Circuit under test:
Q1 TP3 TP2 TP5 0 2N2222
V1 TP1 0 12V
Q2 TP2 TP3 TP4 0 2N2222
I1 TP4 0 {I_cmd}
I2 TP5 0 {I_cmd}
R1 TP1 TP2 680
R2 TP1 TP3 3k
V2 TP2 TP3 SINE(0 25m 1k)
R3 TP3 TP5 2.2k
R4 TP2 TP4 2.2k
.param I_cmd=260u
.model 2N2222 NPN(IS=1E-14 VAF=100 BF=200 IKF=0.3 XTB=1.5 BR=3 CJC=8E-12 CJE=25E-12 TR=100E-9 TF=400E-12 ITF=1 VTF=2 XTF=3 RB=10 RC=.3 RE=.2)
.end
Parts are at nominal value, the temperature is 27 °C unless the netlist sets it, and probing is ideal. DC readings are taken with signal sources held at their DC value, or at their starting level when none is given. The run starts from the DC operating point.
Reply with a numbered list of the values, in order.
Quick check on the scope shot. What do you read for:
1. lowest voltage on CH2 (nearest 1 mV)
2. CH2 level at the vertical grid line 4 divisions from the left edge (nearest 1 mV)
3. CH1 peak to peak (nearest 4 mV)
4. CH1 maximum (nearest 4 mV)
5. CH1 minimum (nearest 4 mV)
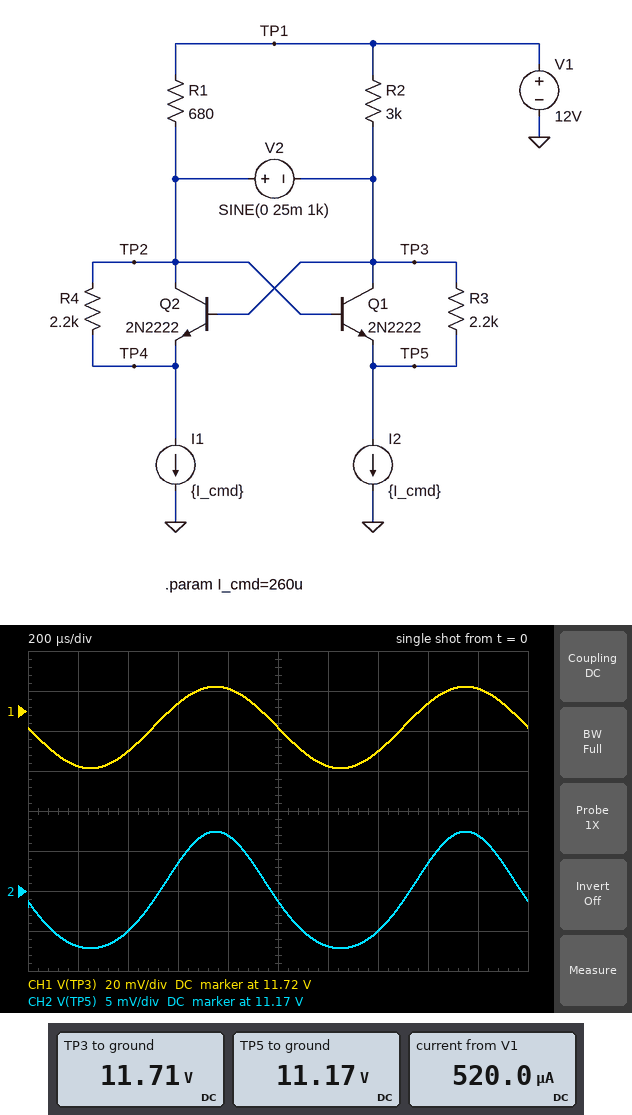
1. 11.163 V
2. 11.177 V
3. 40 mV
4. 11.732 V
5. 11.692 V
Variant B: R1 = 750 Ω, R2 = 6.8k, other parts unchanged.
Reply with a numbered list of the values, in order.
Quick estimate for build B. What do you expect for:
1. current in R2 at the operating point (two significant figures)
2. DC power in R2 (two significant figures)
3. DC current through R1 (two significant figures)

1. 52 µA
2. 18 µW
3. 470 µA
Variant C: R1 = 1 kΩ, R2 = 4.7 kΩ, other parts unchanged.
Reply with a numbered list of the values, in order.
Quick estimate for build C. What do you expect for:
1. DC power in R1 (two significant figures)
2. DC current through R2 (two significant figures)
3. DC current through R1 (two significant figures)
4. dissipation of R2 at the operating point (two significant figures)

1. 180 µW
2. 91 µA
3. 430 µA
4. 39 µW
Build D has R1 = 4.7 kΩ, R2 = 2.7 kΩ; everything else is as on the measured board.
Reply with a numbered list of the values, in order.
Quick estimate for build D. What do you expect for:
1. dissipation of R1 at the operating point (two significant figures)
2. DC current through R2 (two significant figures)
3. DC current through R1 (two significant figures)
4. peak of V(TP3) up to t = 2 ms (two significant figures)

1. 170 µW
2. 330 µA
3. 190 µA
4. 11 V
